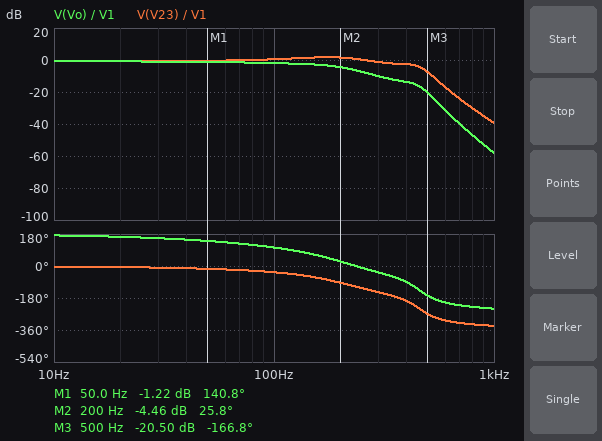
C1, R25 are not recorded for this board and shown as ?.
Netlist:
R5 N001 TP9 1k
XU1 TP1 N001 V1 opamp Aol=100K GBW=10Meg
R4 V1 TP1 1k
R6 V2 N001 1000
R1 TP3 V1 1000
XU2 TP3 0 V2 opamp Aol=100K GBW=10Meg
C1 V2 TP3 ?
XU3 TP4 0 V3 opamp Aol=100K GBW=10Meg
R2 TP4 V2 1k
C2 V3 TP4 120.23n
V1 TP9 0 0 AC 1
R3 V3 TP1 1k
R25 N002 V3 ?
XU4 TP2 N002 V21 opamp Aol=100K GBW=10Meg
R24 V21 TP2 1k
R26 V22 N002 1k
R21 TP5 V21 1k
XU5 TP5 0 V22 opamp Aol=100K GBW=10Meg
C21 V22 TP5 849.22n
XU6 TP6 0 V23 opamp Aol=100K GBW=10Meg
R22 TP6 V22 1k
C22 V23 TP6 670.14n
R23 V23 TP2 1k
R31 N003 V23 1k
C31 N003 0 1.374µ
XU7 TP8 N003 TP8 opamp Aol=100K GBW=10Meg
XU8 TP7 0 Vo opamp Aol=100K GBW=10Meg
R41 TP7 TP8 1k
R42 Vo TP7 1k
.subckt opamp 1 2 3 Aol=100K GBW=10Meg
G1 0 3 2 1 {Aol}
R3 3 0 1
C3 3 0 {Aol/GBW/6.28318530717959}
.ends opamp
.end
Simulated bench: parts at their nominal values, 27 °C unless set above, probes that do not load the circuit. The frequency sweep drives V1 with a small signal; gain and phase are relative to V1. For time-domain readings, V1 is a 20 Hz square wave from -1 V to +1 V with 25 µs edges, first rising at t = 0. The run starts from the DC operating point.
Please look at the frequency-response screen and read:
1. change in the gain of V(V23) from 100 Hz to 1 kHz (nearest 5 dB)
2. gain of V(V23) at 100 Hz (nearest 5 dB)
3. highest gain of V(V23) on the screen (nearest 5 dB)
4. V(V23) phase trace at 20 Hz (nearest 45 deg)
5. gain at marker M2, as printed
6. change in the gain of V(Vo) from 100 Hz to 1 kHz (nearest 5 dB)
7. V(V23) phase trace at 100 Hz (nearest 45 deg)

-40 dB
0 dB
0 dB
0 deg
-4.46 dB
-55 dB
-45 deg
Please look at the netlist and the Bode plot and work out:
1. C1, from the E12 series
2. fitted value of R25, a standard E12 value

1 µF
1.2 kΩ
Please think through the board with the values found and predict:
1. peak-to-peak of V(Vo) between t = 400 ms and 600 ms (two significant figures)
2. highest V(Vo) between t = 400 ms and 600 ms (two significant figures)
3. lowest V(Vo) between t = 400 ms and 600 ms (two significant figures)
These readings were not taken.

1.8 V
910 mV
-910 mV
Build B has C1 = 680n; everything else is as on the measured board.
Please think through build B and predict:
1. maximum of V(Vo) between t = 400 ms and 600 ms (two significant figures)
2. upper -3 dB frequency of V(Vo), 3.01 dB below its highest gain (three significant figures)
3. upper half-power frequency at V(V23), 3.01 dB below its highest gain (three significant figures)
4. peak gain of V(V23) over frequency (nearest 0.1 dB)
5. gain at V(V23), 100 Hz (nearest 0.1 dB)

910 mV
174 Hz
271 Hz
1.3 dB
0.3 dB
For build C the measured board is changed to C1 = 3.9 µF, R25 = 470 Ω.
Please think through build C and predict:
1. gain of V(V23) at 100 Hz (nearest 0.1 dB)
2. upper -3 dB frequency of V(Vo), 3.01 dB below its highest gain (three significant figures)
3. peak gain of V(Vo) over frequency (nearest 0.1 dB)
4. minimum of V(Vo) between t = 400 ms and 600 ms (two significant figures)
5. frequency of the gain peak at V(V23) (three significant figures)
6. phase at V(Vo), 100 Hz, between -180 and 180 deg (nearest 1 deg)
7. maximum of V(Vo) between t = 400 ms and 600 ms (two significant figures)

6.1 dB
243 Hz
14.9 dB
-2.8 V
227 Hz
115 deg
2.8 V
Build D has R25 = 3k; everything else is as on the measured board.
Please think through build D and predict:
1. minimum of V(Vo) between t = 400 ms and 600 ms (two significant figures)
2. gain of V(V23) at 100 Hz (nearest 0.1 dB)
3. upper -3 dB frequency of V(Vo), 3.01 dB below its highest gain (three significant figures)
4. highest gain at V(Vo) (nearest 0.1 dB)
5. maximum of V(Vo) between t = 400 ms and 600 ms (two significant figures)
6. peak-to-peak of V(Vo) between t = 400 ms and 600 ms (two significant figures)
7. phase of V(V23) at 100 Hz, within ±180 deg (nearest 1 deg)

-500 mV
-5.6 dB
127 Hz
-6.0 dB
500 mV
1.0 V
-44 deg
